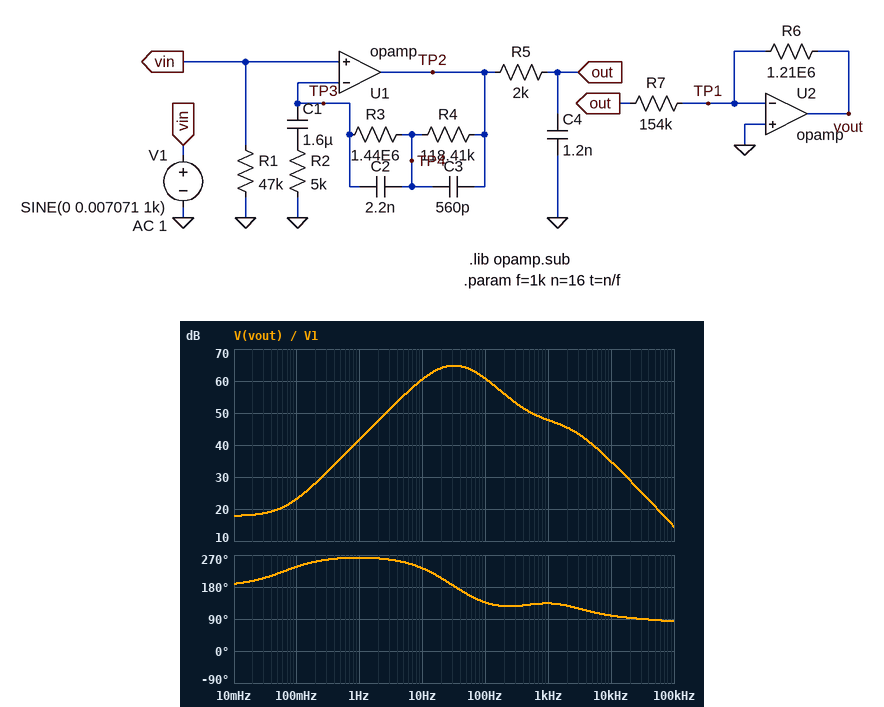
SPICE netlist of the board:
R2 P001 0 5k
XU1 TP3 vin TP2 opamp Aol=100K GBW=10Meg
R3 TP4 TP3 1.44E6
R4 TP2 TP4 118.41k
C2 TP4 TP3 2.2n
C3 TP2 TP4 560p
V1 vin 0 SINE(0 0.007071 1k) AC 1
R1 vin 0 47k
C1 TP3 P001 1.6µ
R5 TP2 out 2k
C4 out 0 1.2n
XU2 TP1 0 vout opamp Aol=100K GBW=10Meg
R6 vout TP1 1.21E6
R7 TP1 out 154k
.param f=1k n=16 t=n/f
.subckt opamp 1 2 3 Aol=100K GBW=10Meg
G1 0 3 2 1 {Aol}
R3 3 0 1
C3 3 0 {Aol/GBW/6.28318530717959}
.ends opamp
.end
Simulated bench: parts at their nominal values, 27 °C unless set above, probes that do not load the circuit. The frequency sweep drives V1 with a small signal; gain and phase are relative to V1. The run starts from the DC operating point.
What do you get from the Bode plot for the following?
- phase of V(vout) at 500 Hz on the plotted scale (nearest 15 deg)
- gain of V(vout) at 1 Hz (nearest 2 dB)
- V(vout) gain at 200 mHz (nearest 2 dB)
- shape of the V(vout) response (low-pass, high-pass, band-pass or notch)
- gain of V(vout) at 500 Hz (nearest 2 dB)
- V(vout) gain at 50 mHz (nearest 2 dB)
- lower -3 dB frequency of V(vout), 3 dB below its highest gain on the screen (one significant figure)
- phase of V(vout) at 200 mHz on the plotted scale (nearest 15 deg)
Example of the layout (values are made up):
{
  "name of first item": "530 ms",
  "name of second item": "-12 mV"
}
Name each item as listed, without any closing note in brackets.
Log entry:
{
  "phase of V(vout) at 500 Hz on the plotted scale": "135 deg",
  "gain of V(vout) at 1 Hz": "42 dB",
  "V(vout) gain at 200 mHz": "28 dB",
  "shape of the V(vout) response": "band-pass",
  "gain of V(vout) at 500 Hz": "50 dB",
  "V(vout) gain at 50 mHz": "20 dB",
  "lower -3 dB frequency of V(vout), 3 dB below its highest gain on the screen": "10 Hz",
  "phase of V(vout) at 200 mHz on the plotted scale": "255 deg"
}
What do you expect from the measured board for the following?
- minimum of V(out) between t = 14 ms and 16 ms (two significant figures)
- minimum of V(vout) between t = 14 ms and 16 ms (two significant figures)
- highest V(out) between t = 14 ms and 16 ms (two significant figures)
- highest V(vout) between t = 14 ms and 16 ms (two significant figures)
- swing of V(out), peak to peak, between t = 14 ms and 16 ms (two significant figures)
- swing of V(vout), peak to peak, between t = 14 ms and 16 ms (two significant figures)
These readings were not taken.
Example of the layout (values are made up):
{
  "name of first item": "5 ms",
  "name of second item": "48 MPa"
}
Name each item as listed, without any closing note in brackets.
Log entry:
{
  "minimum of V(out) between t = 14 ms and 16 ms": "-230 mV",
  "minimum of V(vout) between t = 14 ms and 16 ms": "-1.7 V",
  "highest V(out) between t = 14 ms and 16 ms": "210 mV",
  "highest V(vout) between t = 14 ms and 16 ms": "1.8 V",
  "swing of V(out), peak to peak, between t = 14 ms and 16 ms": "440 mV",
  "swing of V(vout), peak to peak, between t = 14 ms and 16 ms": "3.5 V"
}
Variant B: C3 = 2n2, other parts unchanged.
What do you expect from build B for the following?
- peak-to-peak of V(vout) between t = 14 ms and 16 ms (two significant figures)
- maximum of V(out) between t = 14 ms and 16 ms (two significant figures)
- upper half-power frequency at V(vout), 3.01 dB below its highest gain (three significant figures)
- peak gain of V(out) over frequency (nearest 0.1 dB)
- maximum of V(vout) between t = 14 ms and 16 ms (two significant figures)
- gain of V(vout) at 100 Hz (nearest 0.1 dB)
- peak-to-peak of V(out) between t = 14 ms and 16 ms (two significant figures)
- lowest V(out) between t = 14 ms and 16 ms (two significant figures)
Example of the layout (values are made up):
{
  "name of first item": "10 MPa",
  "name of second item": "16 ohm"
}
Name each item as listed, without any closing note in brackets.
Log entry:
{
  "peak-to-peak of V(vout) between t = 14 ms and 16 ms": "2.9 V",
  "maximum of V(out) between t = 14 ms and 16 ms": "170 mV",
  "upper half-power frequency at V(vout), 3.01 dB below its highest gain": "84.7 Hz",
  "peak gain of V(out) over frequency": "46.9 dB",
  "maximum of V(vout) between t = 14 ms and 16 ms": "1.5 V",
  "gain of V(vout) at 100 Hz": "60.8 dB",
  "peak-to-peak of V(out) between t = 14 ms and 16 ms": "370 mV",
  "lowest V(out) between t = 14 ms and 16 ms": "-190 mV"
}
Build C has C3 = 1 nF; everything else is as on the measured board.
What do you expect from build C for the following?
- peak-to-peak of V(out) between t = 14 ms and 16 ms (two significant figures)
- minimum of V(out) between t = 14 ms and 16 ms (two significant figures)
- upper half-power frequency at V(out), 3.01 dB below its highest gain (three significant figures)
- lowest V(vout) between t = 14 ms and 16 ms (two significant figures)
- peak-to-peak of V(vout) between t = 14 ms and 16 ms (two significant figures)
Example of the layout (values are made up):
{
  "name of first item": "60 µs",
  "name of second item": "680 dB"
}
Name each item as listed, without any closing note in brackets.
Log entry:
{
  "peak-to-peak of V(out) between t = 14 ms and 16 ms": "430 mV",
  "minimum of V(out) between t = 14 ms and 16 ms": "-220 mV",
  "upper half-power frequency at V(out), 3.01 dB below its highest gain": "83.9 Hz",
  "lowest V(vout) between t = 14 ms and 16 ms": "-1.6 V",
  "peak-to-peak of V(vout) between t = 14 ms and 16 ms": "3.4 V"
}
